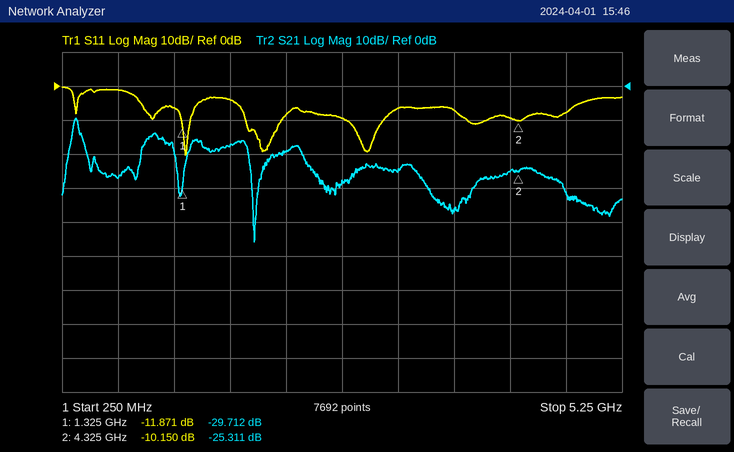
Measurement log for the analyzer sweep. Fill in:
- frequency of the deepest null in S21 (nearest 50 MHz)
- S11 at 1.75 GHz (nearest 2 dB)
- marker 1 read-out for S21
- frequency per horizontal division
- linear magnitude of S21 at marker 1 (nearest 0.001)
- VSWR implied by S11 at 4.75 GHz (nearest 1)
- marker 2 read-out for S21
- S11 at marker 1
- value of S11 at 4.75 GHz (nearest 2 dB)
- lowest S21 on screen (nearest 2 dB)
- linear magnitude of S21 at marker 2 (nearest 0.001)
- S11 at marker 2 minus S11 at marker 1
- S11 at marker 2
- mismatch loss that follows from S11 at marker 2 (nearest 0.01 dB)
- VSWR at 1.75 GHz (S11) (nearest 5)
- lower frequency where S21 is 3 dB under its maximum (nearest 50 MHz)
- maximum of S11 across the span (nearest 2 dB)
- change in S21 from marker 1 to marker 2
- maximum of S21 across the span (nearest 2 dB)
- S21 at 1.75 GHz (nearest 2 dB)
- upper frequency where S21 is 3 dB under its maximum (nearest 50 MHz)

1.95 GHz
-4 dB
-29.712 dB
500 MHz
0.033
2
-25.311 dB
-11.871 dB
-8 dB
-46 dB
0.054
1.721 dB
-10.150 dB
0.44 dB
5
350 MHz
0 dB
4.401 dB
-10 dB
-18 dB
400 MHz
